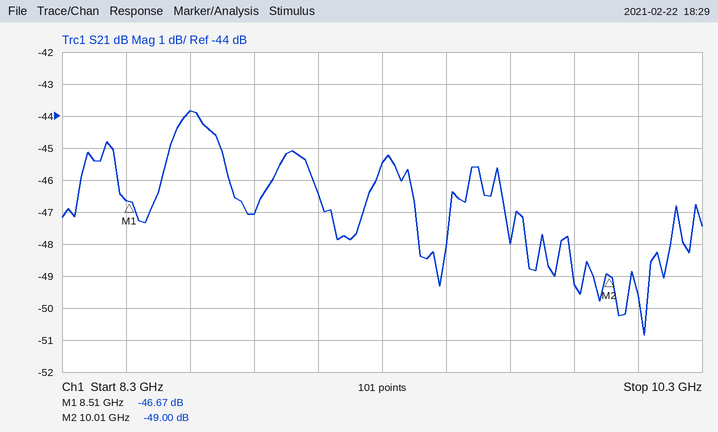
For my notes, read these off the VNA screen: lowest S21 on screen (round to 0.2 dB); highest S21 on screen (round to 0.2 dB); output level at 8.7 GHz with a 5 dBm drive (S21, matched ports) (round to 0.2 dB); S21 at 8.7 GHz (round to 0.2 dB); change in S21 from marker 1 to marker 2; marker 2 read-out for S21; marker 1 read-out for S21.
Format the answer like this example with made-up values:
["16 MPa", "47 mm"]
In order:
["-50.8 dB", "-43.8 dB", "-38.8 dBm", "-43.8 dB", "-2.33 dB", "-49.00 dB", "-46.67 dB"]
